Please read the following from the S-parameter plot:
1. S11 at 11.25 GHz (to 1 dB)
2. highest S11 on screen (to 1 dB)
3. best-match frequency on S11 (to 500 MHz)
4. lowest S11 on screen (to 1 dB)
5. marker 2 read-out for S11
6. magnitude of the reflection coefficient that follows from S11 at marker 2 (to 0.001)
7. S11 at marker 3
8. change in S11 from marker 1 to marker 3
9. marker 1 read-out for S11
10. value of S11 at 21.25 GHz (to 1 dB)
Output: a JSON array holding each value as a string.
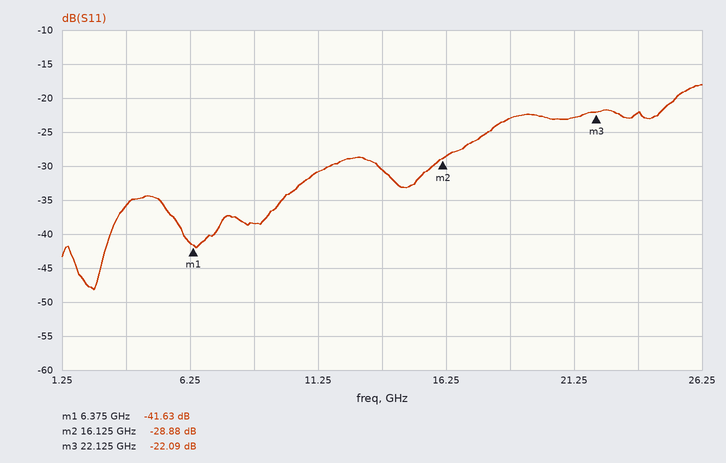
["-31 dB", "-18 dB", "2.5 GHz", "-48 dB", "-28.88 dB", "0.036", "-22.09 dB", "19.54 dB", "-41.63 dB", "-23 dB"]
